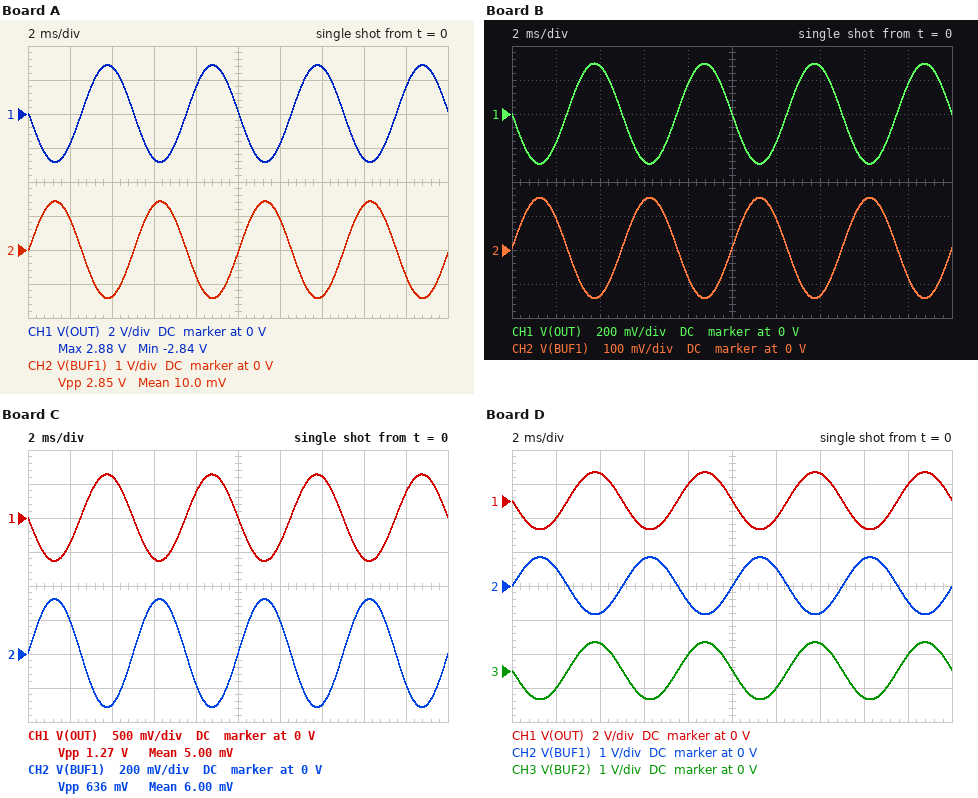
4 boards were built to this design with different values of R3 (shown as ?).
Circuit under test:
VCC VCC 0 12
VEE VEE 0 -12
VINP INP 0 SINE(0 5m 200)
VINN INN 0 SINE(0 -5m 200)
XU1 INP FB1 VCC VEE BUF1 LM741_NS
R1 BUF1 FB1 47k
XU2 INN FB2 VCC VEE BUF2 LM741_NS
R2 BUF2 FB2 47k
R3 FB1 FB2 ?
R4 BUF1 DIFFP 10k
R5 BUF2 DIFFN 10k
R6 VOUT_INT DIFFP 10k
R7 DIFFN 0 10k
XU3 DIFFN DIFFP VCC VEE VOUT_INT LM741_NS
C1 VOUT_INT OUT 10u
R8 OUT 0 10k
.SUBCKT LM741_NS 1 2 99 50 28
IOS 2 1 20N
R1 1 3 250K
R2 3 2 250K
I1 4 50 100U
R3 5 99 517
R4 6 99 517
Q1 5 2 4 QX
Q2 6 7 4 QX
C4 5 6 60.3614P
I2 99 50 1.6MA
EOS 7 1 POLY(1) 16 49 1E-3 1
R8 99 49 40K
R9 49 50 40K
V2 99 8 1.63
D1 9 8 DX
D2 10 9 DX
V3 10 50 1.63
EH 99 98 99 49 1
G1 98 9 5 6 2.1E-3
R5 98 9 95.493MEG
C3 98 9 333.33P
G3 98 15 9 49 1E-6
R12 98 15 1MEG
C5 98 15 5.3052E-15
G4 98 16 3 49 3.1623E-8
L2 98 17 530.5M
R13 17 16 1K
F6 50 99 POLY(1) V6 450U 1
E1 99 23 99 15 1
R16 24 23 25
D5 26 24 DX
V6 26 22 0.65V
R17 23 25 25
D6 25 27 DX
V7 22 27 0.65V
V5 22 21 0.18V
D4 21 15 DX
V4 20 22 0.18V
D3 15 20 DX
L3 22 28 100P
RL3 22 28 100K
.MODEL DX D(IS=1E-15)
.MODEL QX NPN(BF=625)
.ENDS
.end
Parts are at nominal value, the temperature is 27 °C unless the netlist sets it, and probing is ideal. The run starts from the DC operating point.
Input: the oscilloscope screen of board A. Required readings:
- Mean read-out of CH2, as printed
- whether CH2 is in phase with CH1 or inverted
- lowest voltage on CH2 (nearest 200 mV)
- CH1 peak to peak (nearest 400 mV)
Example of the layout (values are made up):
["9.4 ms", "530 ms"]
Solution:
["10.0 mV", "inverted", "-1.4 V", "5.6 V"]
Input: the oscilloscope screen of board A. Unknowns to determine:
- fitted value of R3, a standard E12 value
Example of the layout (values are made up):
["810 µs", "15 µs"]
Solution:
["330 Ω"]
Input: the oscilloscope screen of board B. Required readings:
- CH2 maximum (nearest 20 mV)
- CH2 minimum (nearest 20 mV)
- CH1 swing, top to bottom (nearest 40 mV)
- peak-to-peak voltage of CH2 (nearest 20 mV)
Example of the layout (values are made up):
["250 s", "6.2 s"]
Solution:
["160 mV", "-140 mV", "600 mV", "300 mV"]
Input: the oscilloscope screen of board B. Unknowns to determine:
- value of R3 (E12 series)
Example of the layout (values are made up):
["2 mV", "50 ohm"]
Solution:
["3.3 kΩ"]
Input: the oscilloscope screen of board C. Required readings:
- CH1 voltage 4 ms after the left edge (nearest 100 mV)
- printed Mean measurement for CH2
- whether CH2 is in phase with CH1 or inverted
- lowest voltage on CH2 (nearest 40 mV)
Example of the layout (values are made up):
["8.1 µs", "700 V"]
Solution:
["600 mV", "6.00 mV", "inverted", "-320 mV"]
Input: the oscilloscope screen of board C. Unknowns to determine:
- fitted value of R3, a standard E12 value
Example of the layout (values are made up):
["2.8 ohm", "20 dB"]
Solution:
["1.5 kΩ"]
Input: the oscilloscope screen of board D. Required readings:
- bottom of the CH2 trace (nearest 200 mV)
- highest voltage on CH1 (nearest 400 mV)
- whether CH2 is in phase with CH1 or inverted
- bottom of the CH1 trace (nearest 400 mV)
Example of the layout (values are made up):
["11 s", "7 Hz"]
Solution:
["-800 mV", "1.6 V", "inverted", "-1.6 V"]
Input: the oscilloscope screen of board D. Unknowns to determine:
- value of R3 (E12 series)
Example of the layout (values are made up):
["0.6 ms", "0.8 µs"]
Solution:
["560 Ω"]
